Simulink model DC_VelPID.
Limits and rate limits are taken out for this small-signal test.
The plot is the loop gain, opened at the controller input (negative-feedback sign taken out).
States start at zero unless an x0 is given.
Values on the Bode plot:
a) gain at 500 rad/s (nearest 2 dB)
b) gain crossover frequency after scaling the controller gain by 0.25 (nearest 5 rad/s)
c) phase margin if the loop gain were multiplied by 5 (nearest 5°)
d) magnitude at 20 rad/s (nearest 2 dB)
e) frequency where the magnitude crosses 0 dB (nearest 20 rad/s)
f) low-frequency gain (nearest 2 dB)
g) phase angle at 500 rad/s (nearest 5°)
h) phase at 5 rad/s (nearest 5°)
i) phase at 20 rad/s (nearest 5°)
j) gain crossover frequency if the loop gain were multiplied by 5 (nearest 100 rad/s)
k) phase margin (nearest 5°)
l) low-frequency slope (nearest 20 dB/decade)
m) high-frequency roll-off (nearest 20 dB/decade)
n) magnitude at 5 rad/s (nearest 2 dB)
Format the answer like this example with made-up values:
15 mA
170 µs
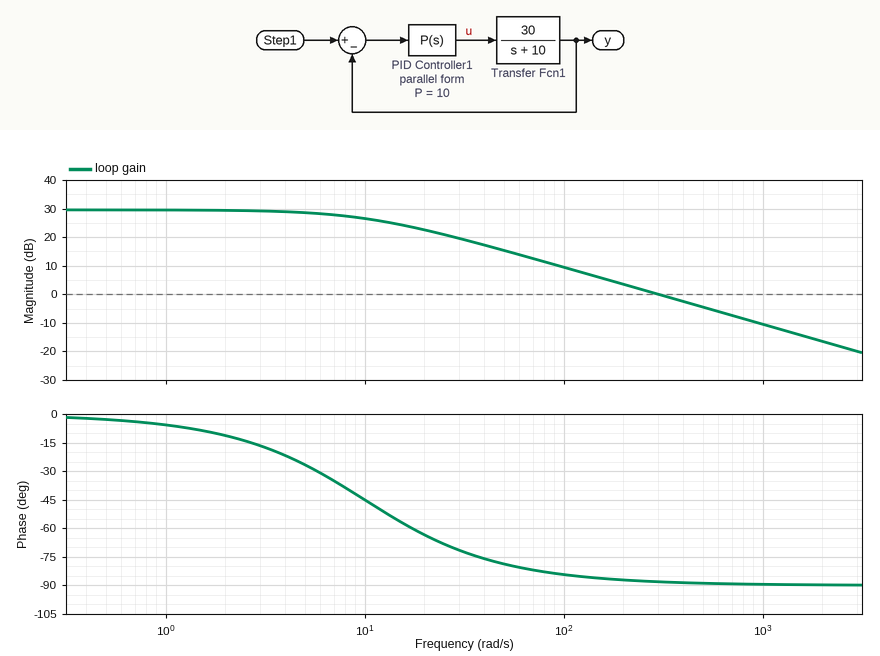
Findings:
-4 dB
75 rad/s
90°
22 dB
300 rad/s
30 dB
-90°
-25°
-65°
1500 rad/s
90°
0 dB/decade
-20 dB/decade
28 dB
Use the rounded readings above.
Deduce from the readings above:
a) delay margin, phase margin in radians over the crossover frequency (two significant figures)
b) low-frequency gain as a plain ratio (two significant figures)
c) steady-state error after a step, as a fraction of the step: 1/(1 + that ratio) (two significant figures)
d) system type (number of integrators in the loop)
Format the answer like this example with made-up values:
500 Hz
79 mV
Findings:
0.0052 s
32
0.030
0
